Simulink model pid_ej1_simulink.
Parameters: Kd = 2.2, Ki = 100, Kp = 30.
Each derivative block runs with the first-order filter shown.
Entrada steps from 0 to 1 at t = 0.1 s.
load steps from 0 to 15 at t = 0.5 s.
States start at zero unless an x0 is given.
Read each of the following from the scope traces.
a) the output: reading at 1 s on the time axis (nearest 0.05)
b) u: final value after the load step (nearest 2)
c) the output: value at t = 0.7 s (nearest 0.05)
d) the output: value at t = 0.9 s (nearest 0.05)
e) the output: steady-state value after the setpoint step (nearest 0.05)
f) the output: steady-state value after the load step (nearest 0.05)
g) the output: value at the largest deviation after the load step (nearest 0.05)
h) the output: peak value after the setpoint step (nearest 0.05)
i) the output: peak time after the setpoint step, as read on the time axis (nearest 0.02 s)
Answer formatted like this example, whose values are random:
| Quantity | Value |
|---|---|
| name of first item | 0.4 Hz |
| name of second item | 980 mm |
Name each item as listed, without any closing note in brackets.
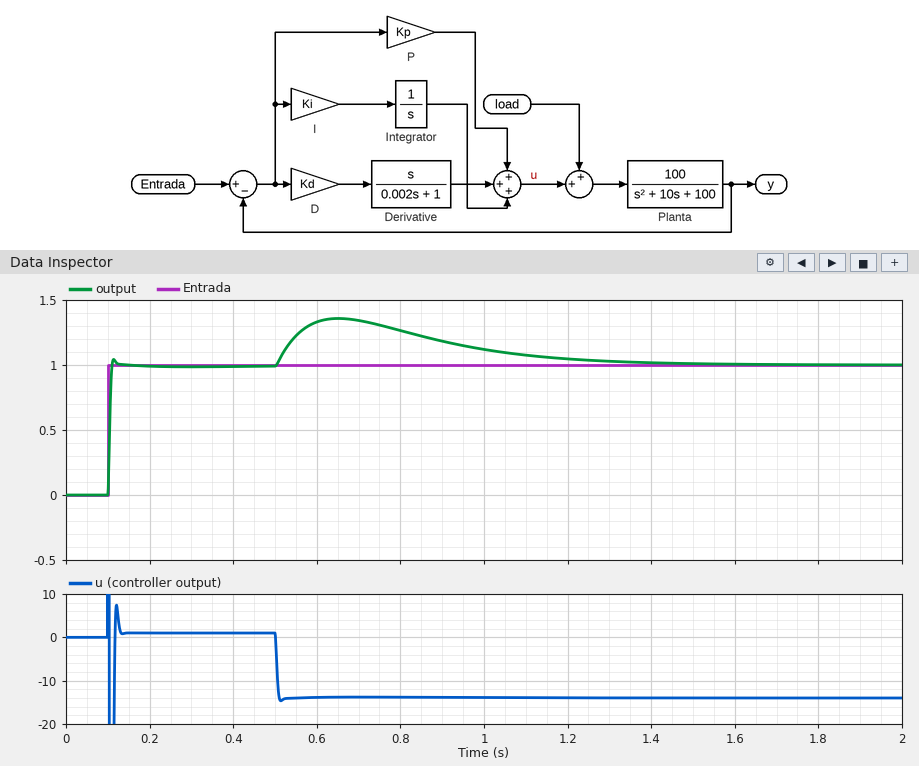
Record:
| Quantity | Value |
|---|---|
| the output: reading at 1 s on the time axis | 1.10 |
| u: final value after the load step | -14 |
| the output: value at t = 0.7 s | 1.35 |
| the output: value at t = 0.9 s | 1.20 |
| the output: steady-state value after the setpoint step | 1.00 |
| the output: steady-state value after the load step | 1.00 |
| the output: value at the largest deviation after the load step | 1.35 |
| the output: peak value after the setpoint step | 1.05 |
| the output: peak time after the setpoint step, as read on the time axis | 0.12 s |
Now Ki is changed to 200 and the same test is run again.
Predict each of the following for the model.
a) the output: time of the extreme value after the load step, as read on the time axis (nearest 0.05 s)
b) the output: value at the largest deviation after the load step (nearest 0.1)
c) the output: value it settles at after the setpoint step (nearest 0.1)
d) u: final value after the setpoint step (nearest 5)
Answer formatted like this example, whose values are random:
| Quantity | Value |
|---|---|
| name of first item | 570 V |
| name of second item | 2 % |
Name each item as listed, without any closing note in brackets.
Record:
| Quantity | Value |
|---|---|
| the output: time of the extreme value after the load step, as read on the time axis | 0.60 s |
| the output: value at the largest deviation after the load step | 1.3 |
| the output: value it settles at after the setpoint step | 1.0 |
| u: final value after the setpoint step | 0 |
